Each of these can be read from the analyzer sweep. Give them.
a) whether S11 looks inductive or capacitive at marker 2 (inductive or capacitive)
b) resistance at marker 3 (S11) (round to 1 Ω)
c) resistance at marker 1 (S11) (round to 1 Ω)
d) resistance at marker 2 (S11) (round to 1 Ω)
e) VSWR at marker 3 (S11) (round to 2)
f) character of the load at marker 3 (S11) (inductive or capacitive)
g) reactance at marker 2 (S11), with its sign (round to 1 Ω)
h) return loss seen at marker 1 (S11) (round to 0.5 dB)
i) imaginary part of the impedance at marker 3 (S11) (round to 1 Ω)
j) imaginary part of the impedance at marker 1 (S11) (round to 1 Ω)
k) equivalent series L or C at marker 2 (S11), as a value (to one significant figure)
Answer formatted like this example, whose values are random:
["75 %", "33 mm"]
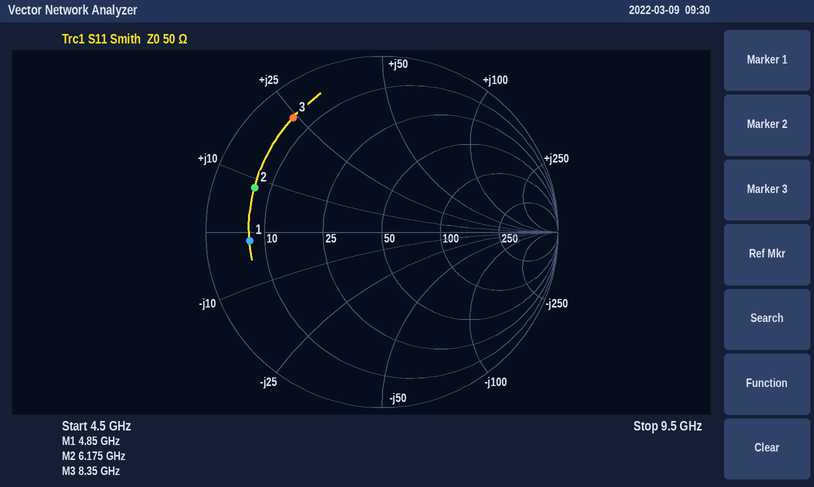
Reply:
["inductive", "6 Ω", "7 Ω", "7 Ω", "10", "inductive", "+8 Ω", "2.5 dB", "+24 Ω", "-2 Ω", "200 pH"]
